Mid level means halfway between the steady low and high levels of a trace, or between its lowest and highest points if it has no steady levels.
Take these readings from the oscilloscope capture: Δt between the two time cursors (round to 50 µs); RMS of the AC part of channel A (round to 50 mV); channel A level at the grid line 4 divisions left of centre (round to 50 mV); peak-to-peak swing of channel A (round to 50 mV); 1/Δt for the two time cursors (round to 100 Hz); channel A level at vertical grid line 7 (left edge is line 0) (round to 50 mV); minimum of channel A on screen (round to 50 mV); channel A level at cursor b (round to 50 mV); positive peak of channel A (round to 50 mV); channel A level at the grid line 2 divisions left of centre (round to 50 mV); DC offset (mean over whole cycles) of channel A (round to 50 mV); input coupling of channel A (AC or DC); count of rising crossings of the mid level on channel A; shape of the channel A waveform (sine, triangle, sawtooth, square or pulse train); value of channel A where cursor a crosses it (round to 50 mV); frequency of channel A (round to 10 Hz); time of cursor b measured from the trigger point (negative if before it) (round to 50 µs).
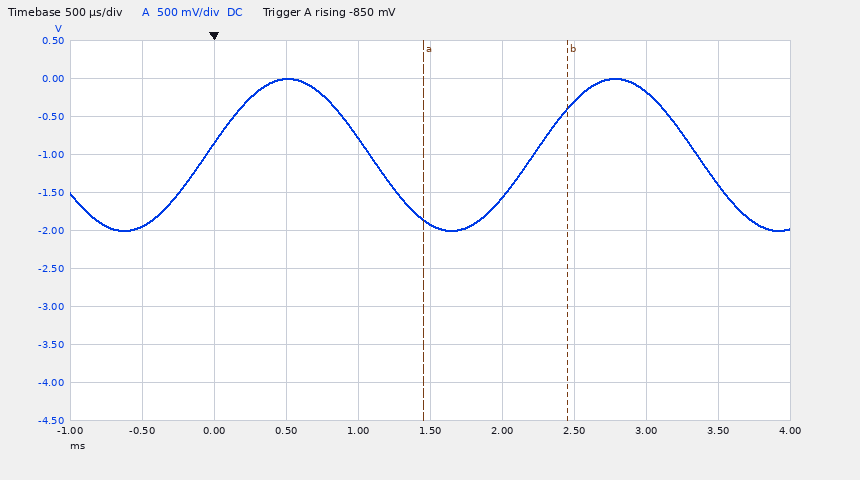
1.00 ms
700 mV
-1.95 V
2.00 V
1.0 kHz
-300 mV
-2.00 V
-400 mV
0 mV
0 mV
-1.00 V
DC
2
sine
-1.85 V
440 Hz
+2.45 ms
